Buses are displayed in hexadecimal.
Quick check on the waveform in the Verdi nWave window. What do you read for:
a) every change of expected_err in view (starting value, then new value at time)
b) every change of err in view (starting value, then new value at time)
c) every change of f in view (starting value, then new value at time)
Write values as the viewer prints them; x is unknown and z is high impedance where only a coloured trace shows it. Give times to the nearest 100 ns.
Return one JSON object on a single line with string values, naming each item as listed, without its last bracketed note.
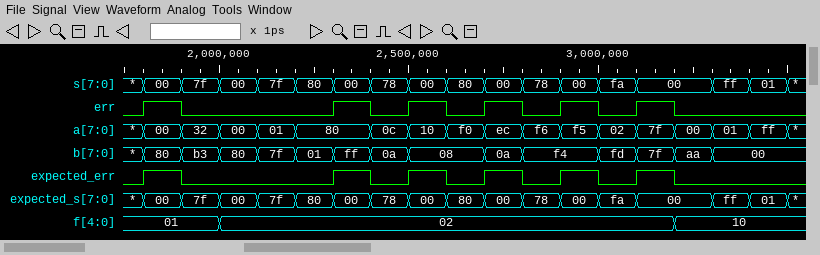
{"every change of expected_err in view": "0, 1 at 1800 ns, 0 at 1900 ns, 1 at 2300 ns, 0 at 2400 ns, 1 at 2500 ns, 0 at 2600 ns, 1 at 2700 ns, 0 at 2800 ns, 1 at 2900 ns, 0 at 3000 ns, 1 at 3100 ns, 0 at 3200 ns", "every change of err in view": "0, 1 at 1800 ns, 0 at 1900 ns, 1 at 2300 ns, 0 at 2400 ns, 1 at 2500 ns, 0 at 2600 ns, 1 at 2700 ns, 0 at 2800 ns, 1 at 2900 ns, 0 at 3000 ns, 1 at 3100 ns, 0 at 3200 ns", "every change of f in view": "01, 02 at 2000 ns, 10 at 3200 ns"}
